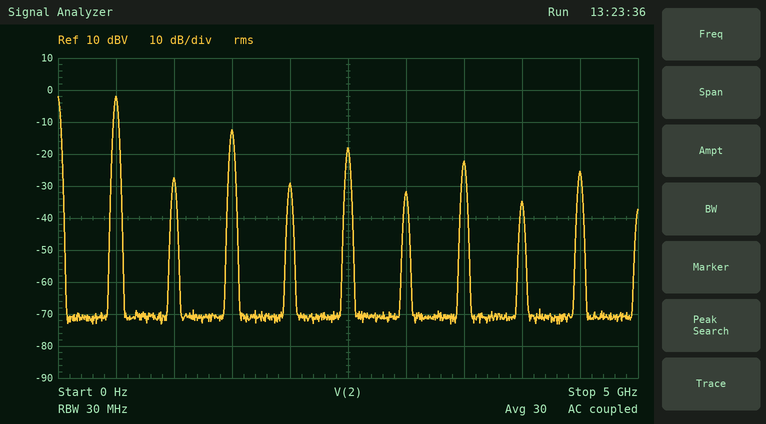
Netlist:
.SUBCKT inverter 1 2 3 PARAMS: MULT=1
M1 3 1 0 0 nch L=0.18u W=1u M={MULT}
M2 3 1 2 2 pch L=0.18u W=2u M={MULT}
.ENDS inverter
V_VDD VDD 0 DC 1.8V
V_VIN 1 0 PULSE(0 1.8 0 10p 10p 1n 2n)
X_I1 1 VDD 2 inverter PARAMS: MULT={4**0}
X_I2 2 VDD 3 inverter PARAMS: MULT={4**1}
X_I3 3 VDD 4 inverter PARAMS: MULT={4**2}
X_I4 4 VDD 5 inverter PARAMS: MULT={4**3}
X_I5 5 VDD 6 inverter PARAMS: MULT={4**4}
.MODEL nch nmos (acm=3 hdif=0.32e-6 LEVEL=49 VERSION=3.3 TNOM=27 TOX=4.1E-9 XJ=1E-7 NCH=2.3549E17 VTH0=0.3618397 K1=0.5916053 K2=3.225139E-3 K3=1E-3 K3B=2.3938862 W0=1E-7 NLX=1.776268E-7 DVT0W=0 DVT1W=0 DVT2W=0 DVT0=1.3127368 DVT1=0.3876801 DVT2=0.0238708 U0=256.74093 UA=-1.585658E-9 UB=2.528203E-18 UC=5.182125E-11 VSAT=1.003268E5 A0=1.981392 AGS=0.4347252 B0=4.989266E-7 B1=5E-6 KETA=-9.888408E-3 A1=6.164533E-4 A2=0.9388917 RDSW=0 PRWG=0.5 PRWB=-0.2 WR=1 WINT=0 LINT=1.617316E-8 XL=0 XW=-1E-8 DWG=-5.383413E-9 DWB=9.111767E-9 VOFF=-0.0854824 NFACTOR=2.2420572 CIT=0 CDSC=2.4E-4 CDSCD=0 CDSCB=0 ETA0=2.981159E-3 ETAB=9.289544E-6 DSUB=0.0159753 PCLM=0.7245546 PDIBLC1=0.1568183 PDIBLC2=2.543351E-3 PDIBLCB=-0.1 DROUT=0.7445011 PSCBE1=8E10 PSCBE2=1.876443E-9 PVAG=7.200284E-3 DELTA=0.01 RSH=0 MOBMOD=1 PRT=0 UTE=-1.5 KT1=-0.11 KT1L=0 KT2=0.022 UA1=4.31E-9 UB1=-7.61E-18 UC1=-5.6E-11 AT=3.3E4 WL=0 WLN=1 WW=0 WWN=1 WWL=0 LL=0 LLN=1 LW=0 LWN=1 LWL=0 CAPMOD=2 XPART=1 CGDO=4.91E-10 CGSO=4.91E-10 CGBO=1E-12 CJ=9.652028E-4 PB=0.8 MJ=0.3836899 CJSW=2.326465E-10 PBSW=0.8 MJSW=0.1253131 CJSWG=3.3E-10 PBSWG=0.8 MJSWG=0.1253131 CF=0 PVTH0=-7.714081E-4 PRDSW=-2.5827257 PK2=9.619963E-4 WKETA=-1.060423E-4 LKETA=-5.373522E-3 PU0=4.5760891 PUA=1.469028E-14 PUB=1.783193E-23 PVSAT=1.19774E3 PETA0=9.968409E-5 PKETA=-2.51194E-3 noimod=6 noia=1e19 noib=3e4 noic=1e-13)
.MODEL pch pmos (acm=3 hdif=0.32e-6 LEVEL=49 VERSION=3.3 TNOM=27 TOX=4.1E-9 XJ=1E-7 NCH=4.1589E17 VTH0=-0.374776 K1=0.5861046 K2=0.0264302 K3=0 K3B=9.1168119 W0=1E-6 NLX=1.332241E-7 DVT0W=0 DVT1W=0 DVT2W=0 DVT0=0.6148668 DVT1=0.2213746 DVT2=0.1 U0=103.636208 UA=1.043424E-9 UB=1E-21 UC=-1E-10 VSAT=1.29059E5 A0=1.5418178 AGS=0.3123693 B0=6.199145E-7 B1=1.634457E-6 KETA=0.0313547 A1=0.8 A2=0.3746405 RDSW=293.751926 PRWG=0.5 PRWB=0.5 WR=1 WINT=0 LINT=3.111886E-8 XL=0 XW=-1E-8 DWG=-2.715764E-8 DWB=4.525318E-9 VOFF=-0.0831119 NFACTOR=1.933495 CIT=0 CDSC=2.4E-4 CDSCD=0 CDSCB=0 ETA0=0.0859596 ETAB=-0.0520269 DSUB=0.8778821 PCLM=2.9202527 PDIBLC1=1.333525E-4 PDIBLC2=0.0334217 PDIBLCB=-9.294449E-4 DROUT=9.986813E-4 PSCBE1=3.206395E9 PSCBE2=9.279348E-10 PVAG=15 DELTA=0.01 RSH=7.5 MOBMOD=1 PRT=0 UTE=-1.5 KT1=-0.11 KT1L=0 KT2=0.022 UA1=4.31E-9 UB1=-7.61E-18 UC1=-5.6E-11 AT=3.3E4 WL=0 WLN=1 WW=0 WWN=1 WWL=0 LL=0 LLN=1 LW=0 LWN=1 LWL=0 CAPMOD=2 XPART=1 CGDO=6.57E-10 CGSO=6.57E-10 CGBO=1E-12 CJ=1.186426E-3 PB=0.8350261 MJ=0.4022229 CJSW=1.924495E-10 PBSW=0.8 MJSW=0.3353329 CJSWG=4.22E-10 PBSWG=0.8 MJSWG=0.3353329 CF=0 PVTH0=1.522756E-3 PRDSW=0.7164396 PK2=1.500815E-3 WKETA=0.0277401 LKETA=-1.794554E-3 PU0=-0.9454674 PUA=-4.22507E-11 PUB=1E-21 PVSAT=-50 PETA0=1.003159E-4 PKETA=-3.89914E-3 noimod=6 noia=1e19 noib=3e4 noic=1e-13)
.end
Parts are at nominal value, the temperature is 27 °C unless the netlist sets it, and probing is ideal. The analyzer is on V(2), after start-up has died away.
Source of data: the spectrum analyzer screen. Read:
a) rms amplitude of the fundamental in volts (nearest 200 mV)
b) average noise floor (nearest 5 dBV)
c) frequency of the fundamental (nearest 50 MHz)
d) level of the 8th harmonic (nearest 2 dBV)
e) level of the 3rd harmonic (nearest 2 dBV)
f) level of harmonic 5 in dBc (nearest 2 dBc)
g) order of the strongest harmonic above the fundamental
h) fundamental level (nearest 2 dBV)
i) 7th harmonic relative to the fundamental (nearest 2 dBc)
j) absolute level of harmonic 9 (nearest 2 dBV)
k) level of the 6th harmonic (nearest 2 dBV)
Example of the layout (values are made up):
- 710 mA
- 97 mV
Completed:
- 800 mV
- -70 dBV
- 500 MHz
- -34 dBV
- -12 dBV
- -16 dBc
- 3
- -2 dBV
- -20 dBc
- -26 dBV
- -32 dBV
